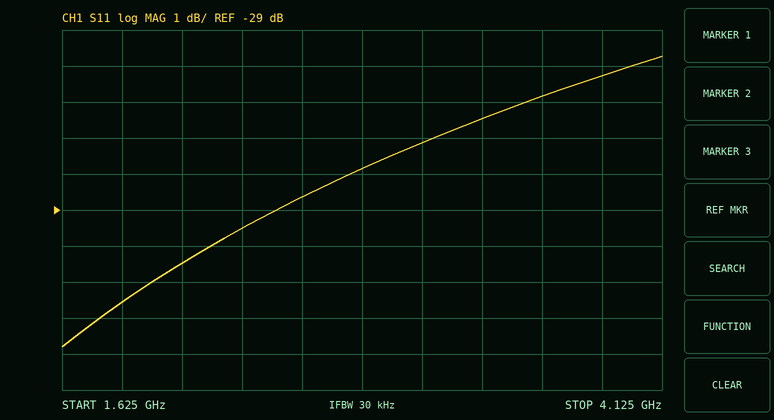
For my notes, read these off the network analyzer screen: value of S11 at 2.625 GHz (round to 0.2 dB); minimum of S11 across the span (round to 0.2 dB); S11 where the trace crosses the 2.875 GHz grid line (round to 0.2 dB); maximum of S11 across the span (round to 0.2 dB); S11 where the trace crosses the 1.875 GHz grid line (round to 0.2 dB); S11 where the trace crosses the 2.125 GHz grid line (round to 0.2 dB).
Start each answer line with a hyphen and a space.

- -28.6 dB
- -32.8 dB
- -27.8 dB
- -24.8 dB
- -31.6 dB
- -30.4 dB
